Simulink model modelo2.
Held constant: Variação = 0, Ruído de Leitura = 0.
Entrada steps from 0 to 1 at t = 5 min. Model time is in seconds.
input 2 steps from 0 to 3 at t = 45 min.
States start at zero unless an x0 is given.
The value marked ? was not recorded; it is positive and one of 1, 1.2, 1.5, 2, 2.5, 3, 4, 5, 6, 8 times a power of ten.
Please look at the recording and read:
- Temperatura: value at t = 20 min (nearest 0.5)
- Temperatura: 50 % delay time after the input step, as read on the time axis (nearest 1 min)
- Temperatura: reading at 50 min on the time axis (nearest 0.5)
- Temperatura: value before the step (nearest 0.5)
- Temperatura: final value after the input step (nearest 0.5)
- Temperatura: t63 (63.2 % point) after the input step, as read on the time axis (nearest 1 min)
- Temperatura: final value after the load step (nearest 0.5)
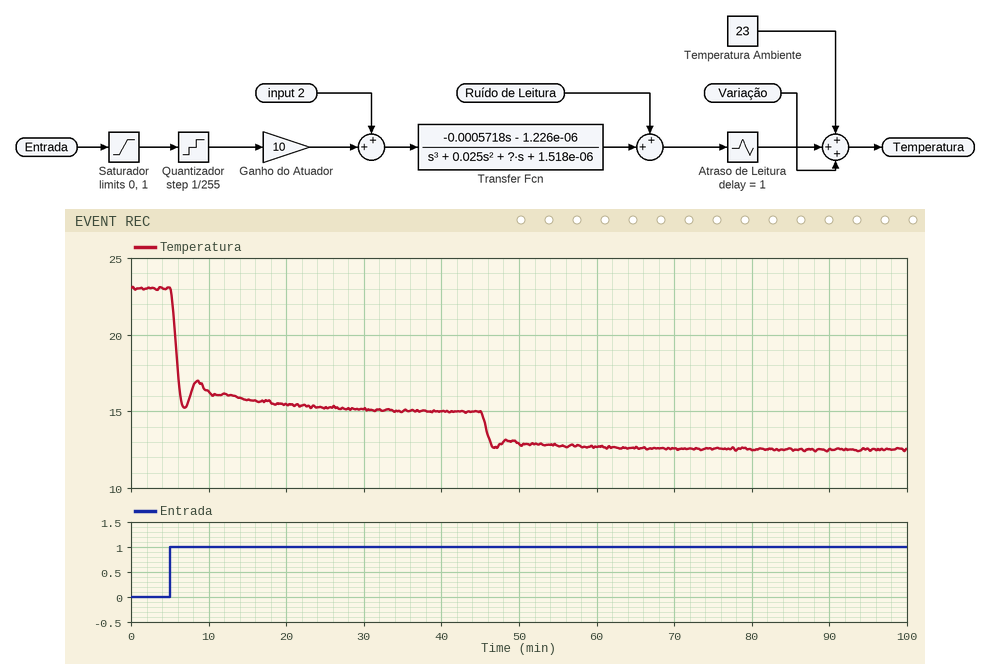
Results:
15.5
6 min
13.0
23.0
15.0
6 min
12.5
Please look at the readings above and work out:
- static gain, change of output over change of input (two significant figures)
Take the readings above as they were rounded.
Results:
-8.0
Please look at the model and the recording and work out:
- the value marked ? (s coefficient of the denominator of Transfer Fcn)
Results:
0.001
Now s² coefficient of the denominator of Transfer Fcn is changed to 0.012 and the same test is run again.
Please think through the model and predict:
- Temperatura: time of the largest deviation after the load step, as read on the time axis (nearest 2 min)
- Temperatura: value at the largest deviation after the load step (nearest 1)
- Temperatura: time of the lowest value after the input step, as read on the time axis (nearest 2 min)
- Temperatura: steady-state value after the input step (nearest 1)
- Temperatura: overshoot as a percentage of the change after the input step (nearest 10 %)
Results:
46 min
12
6 min
15
20 %
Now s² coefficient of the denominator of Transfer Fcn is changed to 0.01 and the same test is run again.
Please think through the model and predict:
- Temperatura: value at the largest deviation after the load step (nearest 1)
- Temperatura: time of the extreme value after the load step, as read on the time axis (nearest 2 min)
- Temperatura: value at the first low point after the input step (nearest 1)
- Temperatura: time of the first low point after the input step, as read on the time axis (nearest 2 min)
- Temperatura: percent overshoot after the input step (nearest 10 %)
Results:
12
46 min
13
6 min
20 %
